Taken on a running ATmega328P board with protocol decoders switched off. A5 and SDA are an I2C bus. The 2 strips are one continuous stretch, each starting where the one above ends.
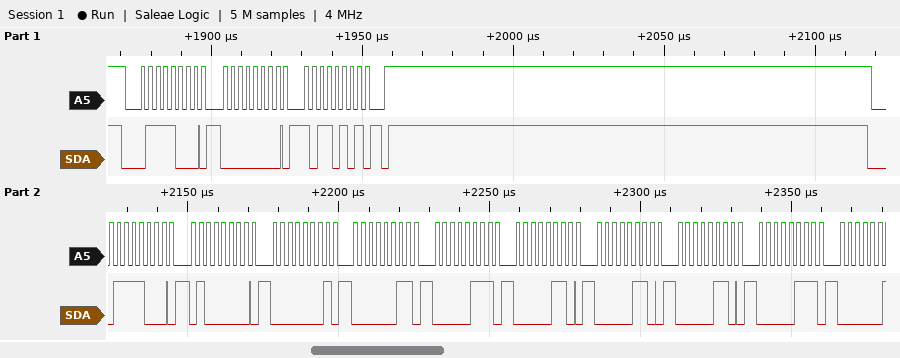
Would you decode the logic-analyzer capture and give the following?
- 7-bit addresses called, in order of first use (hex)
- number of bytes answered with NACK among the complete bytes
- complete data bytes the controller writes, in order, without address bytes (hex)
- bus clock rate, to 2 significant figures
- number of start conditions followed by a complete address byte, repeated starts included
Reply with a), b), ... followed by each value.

a) 0x3C
b) 0
c) 00 B5 40 01 03 07 06 06 06 07
d) 400 kHz
e) 2
